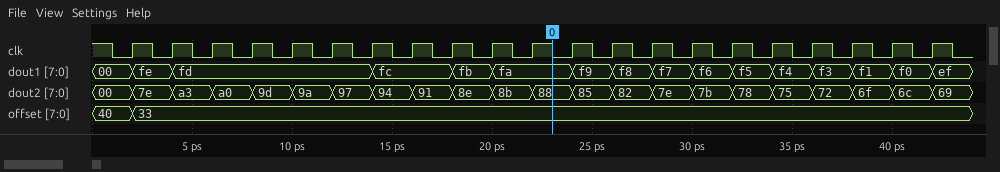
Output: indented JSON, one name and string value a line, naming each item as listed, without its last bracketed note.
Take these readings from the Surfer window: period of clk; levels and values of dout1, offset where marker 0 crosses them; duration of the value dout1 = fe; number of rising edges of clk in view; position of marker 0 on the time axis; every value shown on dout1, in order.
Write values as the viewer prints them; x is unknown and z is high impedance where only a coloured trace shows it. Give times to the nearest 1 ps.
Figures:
{
  "period of clk": "2 ps",
  "levels and values of dout1, offset where marker 0 crosses them": "dout1=fa, offset=33",
  "duration of the value dout1 = fe": "2 ps",
  "number of rising edges of clk in view": "21",
  "position of marker 0 on the time axis": "23 ps",
  "every value shown on dout1, in order": "00, fe, fd, fc, fb, fa, f9, f8, f7, f6, f5, f4, f3, f1, f0, ef"
}
